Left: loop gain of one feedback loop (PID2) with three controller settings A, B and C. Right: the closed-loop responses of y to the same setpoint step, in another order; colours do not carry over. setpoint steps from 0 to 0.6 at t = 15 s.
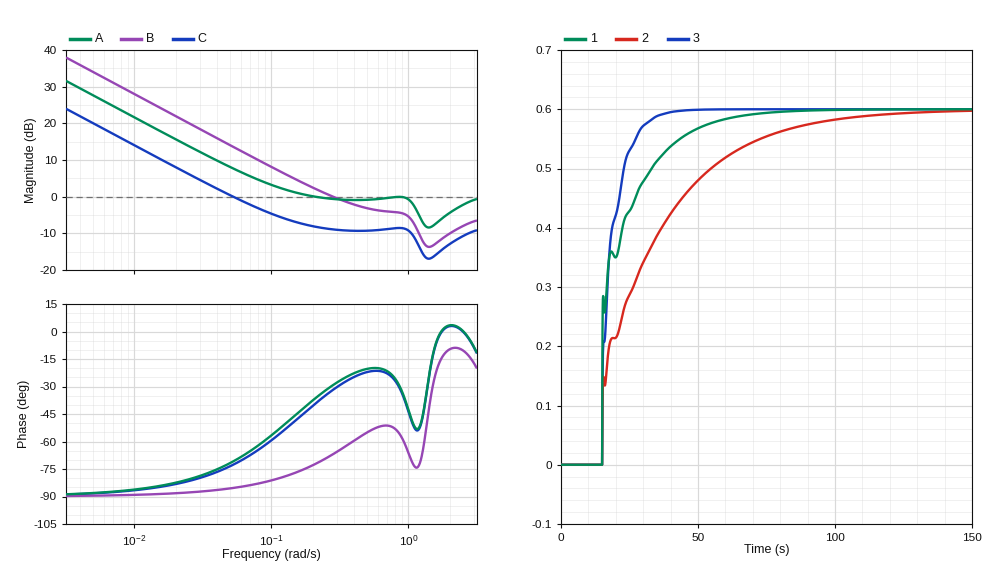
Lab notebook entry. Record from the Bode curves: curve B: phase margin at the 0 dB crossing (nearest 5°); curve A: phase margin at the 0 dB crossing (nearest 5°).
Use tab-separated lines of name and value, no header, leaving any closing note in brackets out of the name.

curve B: phase margin at the 0 dB crossing	115°
curve A: phase margin at the 0 dB crossing	145°
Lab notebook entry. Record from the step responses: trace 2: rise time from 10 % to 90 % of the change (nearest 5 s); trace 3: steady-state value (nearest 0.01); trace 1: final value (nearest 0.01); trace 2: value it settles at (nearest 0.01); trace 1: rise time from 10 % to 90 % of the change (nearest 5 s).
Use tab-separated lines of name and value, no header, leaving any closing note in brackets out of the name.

trace 2: rise time from 10 % to 90 % of the change	55 s
trace 3: steady-state value	0.60
trace 1: final value	0.60
trace 2: value it settles at	0.60
trace 1: rise time from 10 % to 90 % of the change	25 s
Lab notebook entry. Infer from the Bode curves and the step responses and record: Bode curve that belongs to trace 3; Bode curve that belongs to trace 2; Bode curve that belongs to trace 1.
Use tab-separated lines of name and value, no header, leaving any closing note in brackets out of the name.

Bode curve that belongs to trace 3	B
Bode curve that belongs to trace 2	C
Bode curve that belongs to trace 1	A
